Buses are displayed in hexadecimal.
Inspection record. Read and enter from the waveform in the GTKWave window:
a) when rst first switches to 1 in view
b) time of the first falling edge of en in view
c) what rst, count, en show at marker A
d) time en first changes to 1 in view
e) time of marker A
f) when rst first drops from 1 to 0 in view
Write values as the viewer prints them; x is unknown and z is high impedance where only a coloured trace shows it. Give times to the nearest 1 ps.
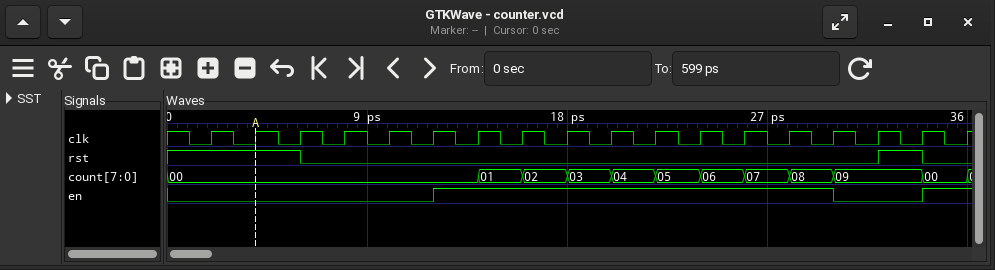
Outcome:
32 ps
30 ps
rst=1, count=00, en=0
12 ps
4 ps
6 ps
